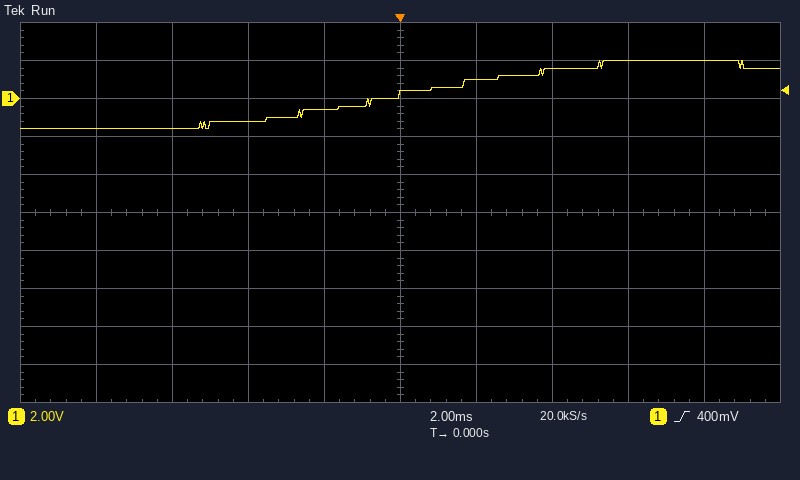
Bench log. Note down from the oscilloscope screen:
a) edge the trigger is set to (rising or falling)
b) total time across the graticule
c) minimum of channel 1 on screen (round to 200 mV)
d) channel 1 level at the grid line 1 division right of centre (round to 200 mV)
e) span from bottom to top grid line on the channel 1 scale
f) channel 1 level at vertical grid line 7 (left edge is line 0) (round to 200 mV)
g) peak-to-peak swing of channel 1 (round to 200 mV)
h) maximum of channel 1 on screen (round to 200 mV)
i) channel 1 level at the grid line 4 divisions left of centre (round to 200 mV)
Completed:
rising
20 ms
-1.6 V
1.0 V
20 V
1.6 V
3.6 V
2.0 V
-1.6 V
